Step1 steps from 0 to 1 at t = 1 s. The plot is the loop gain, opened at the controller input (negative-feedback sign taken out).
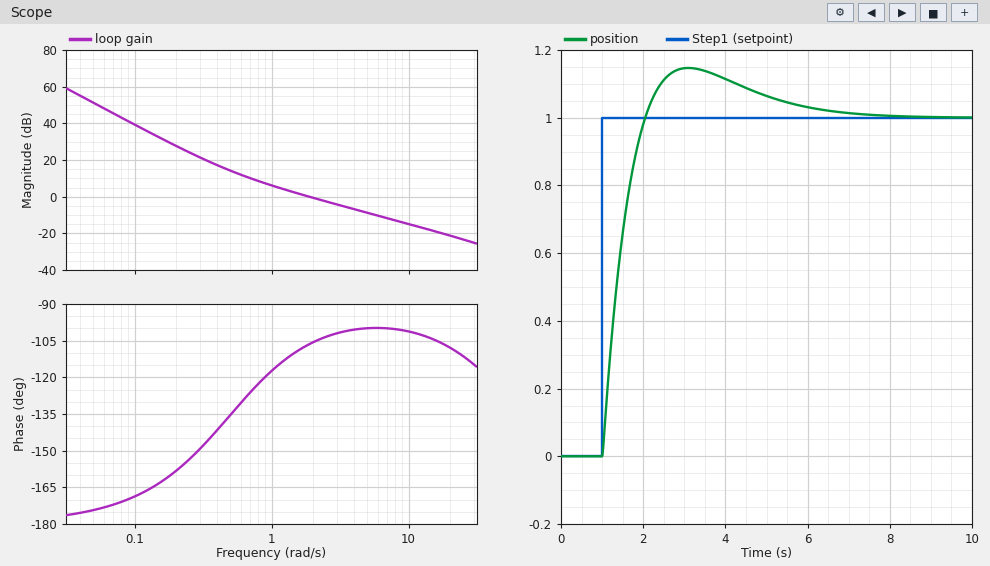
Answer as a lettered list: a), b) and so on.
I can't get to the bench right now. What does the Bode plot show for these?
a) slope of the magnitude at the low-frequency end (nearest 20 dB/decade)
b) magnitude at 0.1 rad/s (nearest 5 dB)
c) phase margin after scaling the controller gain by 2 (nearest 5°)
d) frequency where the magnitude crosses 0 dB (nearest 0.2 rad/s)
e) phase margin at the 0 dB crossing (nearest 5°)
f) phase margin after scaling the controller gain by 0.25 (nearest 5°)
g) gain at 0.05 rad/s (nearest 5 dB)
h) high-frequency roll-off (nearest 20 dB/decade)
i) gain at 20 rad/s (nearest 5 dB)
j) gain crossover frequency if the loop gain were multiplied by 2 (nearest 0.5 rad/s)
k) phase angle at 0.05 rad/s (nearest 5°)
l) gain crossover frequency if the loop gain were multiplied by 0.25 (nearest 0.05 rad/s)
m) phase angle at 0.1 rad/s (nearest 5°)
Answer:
a) -40 dB/decade
b) 40 dB
c) 80°
d) 1.8 rad/s
e) 75°
f) 50°
g) 50 dB
h) -20 dB/decade
i) -20 dB
j) 3.5 rad/s
k) -175°
l) 0.60 rad/s
m) -170°
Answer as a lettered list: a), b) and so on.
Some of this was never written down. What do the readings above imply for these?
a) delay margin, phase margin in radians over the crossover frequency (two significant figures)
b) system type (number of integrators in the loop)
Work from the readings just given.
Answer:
a) 0.73 s
b) 2
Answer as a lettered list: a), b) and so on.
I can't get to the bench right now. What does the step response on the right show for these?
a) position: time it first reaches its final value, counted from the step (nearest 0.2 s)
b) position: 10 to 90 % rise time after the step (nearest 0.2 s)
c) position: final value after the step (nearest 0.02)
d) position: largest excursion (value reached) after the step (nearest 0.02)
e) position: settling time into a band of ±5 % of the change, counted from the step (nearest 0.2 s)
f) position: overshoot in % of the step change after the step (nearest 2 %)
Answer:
a) 1.0 s
b) 0.8 s
c) 1.00
d) 1.14
e) 4.4 s
f) 14 %
